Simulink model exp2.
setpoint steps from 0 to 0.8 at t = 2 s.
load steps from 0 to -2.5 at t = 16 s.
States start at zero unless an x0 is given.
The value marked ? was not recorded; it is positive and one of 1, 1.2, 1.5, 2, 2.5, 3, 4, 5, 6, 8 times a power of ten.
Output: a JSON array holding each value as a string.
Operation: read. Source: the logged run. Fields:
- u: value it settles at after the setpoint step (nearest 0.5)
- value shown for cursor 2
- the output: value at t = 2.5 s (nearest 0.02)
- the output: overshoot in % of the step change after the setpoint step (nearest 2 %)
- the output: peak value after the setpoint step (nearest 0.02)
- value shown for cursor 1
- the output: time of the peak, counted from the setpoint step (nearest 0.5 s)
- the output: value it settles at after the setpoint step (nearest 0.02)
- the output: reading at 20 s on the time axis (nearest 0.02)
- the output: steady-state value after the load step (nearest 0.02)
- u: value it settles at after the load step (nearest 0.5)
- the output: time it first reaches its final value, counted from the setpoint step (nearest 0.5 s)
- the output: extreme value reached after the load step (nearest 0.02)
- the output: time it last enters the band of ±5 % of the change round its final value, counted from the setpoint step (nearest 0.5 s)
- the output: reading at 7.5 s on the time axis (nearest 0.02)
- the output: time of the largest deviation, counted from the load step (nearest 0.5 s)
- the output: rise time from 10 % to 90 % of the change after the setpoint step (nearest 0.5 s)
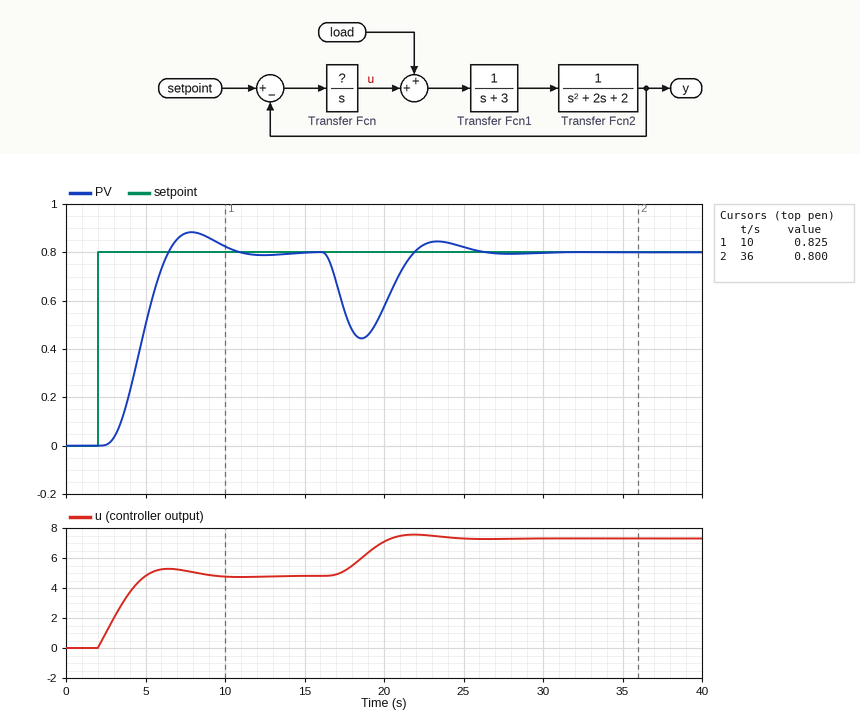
["5.0", "0.800", "0.00", "10 %", "0.88", "0.825", "6.0 s", "0.80", "0.58", "0.80", "7.5", "4.5 s", "0.44", "7.5 s", "0.88", "2.5 s", "2.5 s"]
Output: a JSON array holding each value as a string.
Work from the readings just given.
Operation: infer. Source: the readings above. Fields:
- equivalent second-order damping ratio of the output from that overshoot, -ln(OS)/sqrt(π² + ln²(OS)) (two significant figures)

["0.59"]
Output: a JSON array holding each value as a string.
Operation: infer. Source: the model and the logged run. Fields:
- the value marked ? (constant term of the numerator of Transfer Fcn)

["2.5"]
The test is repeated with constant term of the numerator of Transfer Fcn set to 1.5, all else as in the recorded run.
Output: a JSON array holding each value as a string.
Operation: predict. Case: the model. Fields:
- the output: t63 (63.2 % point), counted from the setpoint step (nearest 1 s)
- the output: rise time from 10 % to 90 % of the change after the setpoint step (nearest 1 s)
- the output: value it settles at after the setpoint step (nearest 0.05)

["4 s", "5 s", "0.80"]
